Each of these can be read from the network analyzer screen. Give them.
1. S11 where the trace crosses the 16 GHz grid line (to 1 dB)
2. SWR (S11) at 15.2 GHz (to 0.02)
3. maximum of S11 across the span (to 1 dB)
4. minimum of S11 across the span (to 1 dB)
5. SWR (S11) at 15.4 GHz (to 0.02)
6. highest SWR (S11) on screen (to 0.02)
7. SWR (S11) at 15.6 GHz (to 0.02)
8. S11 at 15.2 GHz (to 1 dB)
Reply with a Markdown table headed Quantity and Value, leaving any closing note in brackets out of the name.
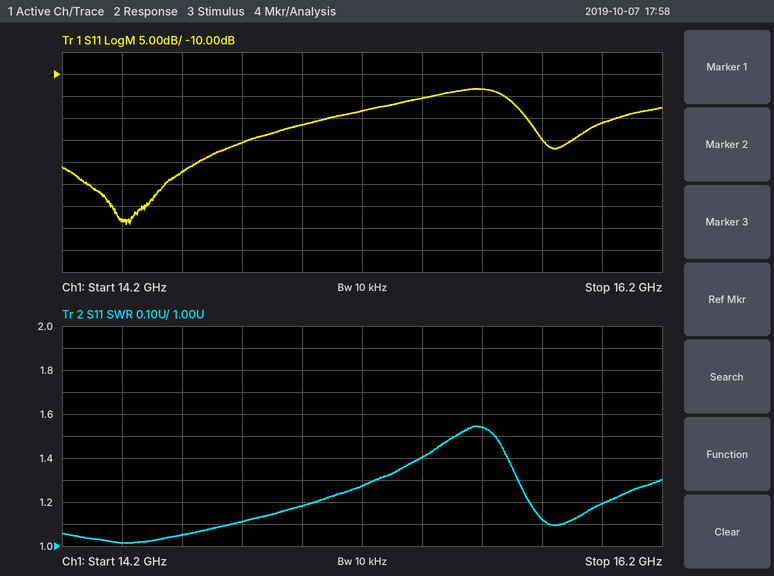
| Quantity | Value |
|---|---|
| S11 where the trace crosses the 16 GHz grid line | -21 dB |
| SWR (S11) at 15.2 GHz | 1.28 |
| maximum of S11 across the span | -13 dB |
| minimum of S11 across the span | -44 dB |
| SWR (S11) at 15.4 GHz | 1.40 |
| highest SWR (S11) on screen | 1.54 |
| SWR (S11) at 15.6 GHz | 1.54 |
| S11 at 15.2 GHz | -18 dB |
